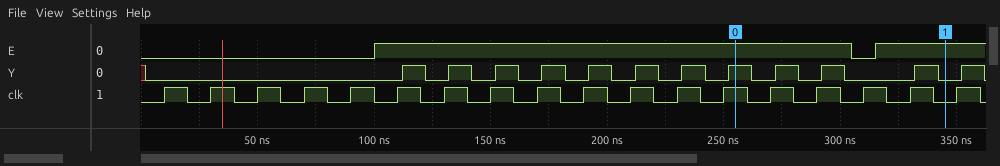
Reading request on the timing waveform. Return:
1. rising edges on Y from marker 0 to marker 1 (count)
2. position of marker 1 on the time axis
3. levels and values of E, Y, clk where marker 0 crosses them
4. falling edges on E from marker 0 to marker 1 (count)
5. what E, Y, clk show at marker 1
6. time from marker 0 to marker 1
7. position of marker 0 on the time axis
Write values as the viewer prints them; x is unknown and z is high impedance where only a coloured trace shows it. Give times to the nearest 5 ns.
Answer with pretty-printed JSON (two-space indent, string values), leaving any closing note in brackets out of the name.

{
  "rising edges on Y from marker 0 to marker 1": "3",
  "position of marker 1 on the time axis": "345 ns",
  "levels and values of E, Y, clk where marker 0 crosses them": "E=1, Y=1, clk=1",
  "falling edges on E from marker 0 to marker 1": "1",
  "what E, Y, clk show at marker 1": "E=1, Y=0, clk=0",
  "time from marker 0 to marker 1": "90 ns",
  "position of marker 0 on the time axis": "255 ns"
}
